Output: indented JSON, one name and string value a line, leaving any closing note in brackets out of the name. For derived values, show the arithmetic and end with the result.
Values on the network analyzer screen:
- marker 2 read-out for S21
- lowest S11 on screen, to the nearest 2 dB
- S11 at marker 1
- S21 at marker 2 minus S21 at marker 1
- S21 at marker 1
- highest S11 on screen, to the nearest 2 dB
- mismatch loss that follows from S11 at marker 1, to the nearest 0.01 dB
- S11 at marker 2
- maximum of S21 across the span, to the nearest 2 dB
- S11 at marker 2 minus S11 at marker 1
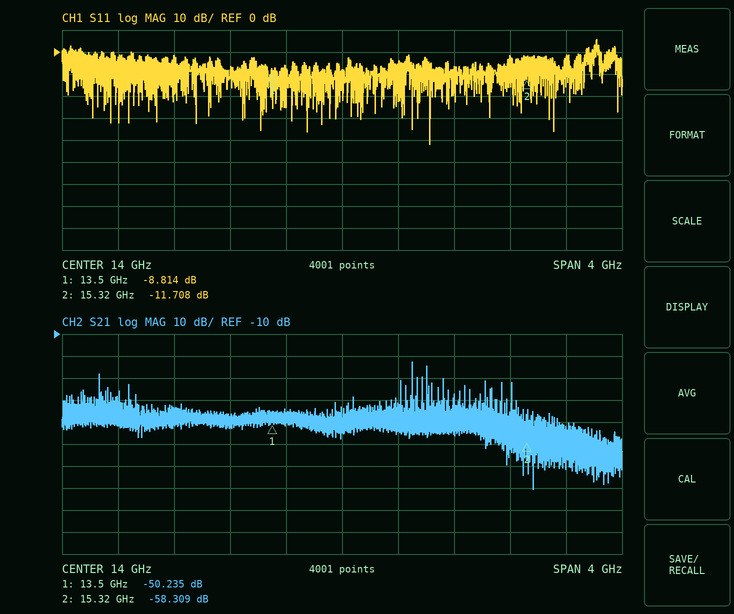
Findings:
{
  "marker 2 read-out for S21": "-58.309 dB",
  "lowest S11 on screen, to the nearest 2 dB": "-42 dB",
  "S11 at marker 1": "-8.814 dB",
  "S21 at marker 2 minus S21 at marker 1": "-58.309 − (-50.235) = -8.074 dB",
  "S21 at marker 1": "-50.235 dB",
  "highest S11 on screen, to the nearest 2 dB": "6 dB",
  "mismatch loss that follows from S11 at marker 1, to the nearest 0.01 dB": "−10 log10(1 − 10^(-8.814/10)) ≈ 0.61 dB",
  "S11 at marker 2": "-11.708 dB",
  "maximum of S21 across the span, to the nearest 2 dB": "-22 dB",
  "S11 at marker 2 minus S11 at marker 1": "-11.708 − (-8.814) = -2.894 dB"
}
